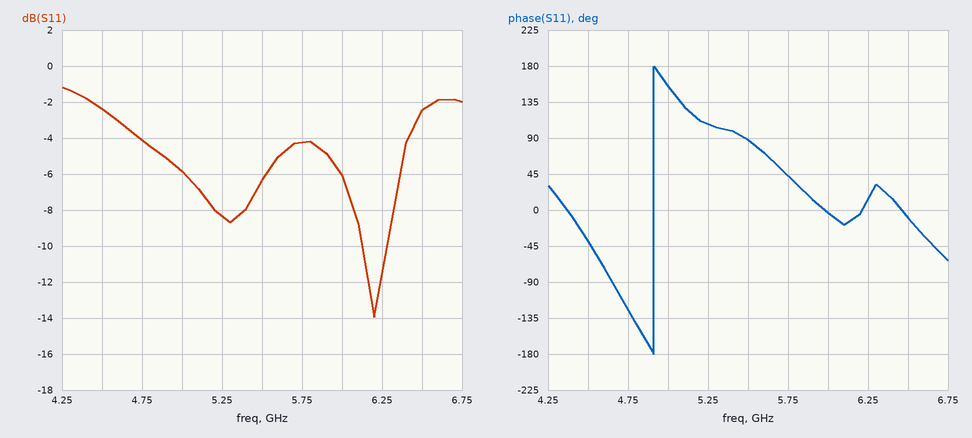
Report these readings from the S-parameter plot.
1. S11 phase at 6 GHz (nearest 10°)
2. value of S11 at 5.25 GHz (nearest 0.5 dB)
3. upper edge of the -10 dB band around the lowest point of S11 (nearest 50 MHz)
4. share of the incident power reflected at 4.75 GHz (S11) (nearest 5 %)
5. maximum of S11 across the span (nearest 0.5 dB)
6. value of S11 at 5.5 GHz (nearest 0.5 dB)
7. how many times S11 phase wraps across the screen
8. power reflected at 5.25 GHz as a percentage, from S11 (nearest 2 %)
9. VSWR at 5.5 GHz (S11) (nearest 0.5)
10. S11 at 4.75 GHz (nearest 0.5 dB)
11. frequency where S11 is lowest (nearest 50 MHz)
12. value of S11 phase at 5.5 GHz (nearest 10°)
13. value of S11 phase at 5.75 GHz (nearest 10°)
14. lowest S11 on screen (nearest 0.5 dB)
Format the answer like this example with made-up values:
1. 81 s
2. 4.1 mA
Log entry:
1. 0°
2. -8.5 dB
3. 6.30 GHz
4. 40 %
5. -1.0 dB
6. -6.5 dB
7. 1
8. 14 %
9. 3.0
10. -4.0 dB
11. 6.20 GHz
12. 90°
13. 40°
14. -14.0 dB
